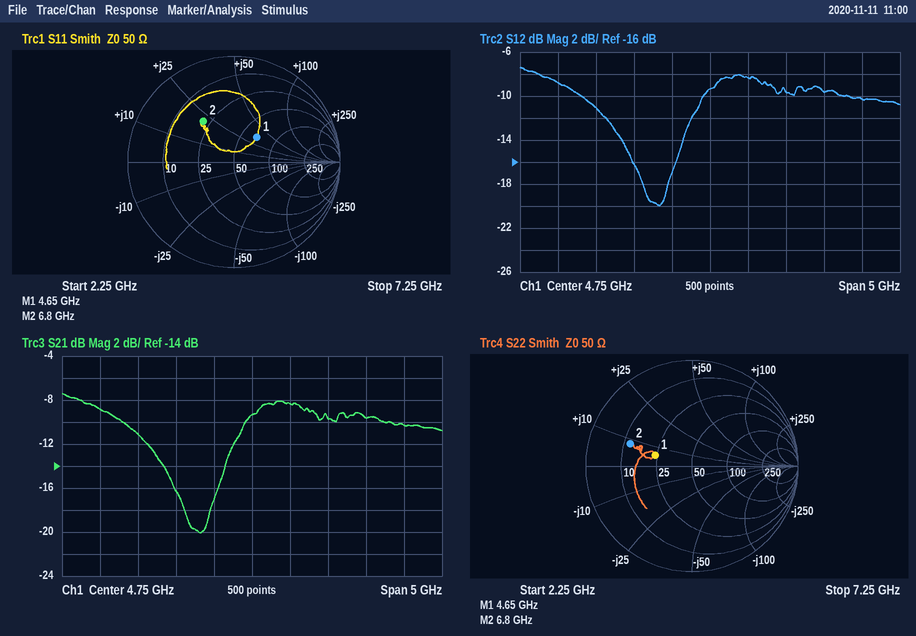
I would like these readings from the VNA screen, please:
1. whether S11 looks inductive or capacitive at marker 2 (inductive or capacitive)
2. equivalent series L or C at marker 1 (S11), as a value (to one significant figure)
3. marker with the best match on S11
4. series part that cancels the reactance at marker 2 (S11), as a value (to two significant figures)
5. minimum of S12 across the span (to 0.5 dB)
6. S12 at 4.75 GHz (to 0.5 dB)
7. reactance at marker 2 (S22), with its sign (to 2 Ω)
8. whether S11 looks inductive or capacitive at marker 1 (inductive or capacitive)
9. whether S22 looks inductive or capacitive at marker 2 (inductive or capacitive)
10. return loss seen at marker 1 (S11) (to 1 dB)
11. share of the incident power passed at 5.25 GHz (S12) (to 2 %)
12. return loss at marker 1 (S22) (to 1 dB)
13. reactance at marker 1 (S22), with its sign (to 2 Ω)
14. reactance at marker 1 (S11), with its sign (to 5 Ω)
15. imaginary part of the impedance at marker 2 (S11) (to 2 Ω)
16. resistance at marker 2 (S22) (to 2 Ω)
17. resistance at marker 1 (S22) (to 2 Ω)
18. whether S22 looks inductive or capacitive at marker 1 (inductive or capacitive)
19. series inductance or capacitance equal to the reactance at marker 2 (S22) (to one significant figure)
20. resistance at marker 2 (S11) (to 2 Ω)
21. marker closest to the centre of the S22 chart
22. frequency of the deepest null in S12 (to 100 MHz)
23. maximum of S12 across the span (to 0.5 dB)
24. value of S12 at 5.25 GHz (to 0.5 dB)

inductive
1 nH
marker 1
1.1 pF
-20.0 dB
-9.5 dB
+8 Ω
inductive
inductive
10 dB
14 %
9 dB
+6 Ω
+35 Ω
+22 Ω
12 Ω
24 Ω
inductive
200 pH
22 Ω
marker 1
4.1 GHz
-7.5 dB
-8.5 dB
